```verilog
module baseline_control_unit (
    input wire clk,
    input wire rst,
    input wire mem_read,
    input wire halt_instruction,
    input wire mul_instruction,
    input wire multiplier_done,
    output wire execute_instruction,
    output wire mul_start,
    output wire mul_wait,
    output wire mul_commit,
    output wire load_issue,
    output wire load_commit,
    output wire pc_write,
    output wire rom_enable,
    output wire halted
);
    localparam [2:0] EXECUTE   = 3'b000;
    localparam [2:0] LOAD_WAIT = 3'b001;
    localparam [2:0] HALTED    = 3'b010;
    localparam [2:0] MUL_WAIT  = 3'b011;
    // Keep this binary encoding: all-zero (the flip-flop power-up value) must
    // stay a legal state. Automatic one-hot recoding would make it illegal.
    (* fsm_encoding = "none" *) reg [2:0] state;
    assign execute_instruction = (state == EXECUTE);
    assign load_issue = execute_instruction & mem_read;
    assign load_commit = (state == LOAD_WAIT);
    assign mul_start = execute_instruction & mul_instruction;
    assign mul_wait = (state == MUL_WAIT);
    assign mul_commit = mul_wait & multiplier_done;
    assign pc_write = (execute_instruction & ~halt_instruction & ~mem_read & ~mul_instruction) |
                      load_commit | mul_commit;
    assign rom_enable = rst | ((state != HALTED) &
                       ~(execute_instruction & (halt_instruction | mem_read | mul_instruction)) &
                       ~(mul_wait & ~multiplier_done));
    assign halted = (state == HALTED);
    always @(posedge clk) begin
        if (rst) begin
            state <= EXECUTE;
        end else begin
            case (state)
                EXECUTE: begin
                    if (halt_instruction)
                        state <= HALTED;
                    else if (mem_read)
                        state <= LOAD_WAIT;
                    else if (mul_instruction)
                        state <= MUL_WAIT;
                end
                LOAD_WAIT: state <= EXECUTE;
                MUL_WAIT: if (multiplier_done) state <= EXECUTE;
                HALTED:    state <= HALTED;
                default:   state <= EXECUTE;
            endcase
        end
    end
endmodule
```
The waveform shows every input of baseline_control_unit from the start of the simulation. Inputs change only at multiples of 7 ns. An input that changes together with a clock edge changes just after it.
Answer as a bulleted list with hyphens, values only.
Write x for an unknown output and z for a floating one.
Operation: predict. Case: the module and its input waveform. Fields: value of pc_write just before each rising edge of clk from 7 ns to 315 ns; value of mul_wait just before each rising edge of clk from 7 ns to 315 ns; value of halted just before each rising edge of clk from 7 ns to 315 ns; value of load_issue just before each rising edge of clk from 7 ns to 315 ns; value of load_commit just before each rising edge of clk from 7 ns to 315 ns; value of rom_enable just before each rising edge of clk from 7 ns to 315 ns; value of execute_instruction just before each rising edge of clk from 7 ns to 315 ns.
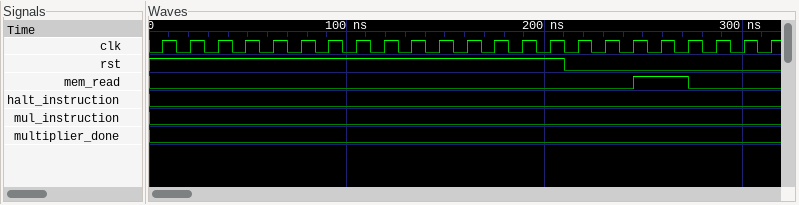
- x 1 1 1 1 1 1 1 1 1 1 1 1 1 1 1 1 1 0 1 1 1 1
- x 0 0 0 0 0 0 0 0 0 0 0 0 0 0 0 0 0 0 0 0 0 0
- x 0 0 0 0 0 0 0 0 0 0 0 0 0 0 0 0 0 0 0 0 0 0
- 0 0 0 0 0 0 0 0 0 0 0 0 0 0 0 0 0 0 1 0 0 0 0
- x 0 0 0 0 0 0 0 0 0 0 0 0 0 0 0 0 0 0 1 0 0 0
- 1 1 1 1 1 1 1 1 1 1 1 1 1 1 1 1 1 1 0 1 1 1 1
- x 1 1 1 1 1 1 1 1 1 1 1 1 1 1 1 1 1 1 0 1 1 1
